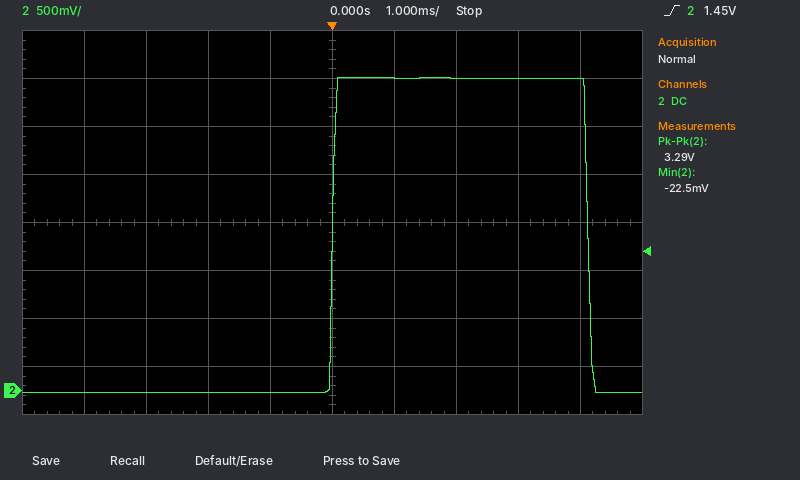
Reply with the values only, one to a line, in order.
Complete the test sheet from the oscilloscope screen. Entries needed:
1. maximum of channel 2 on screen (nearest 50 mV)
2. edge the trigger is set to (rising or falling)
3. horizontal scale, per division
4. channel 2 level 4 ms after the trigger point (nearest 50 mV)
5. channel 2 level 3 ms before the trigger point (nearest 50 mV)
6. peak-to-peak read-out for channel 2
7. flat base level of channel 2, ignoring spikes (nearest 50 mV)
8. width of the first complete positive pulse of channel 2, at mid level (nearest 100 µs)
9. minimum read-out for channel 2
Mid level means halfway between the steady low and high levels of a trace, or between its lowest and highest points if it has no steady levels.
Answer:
3.25 V
rising
1 ms
3.25 V
0 mV
3.29 V
0 mV
4.1 ms
-22.5 mV
